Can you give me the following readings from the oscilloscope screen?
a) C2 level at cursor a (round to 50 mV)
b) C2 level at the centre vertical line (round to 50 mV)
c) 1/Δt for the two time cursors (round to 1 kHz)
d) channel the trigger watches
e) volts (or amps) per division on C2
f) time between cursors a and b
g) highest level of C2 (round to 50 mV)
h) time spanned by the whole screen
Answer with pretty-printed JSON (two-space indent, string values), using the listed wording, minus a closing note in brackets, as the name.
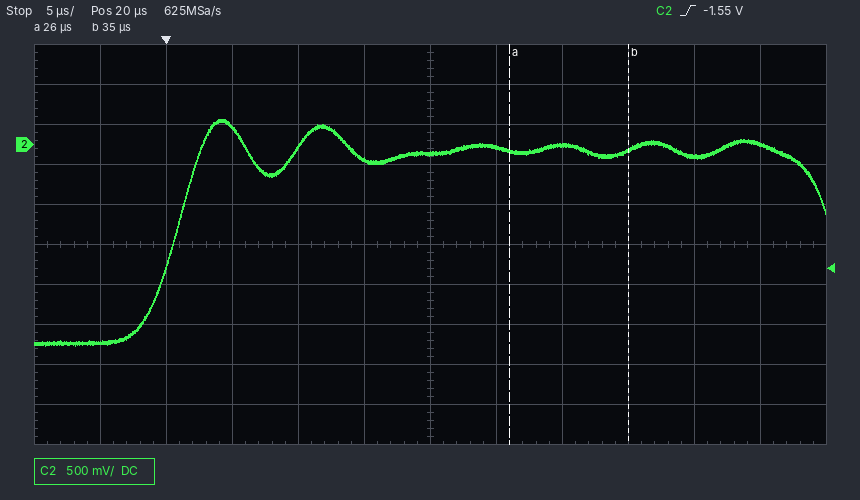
{
  "C2 level at cursor a": "-100 mV",
  "C2 level at the centre vertical line": "-100 mV",
  "1/Δt for the two time cursors": "111 kHz",
  "channel the trigger watches": "C2",
  "volts (or amps) per division on C2": "500 mV",
  "time between cursors a and b": "9.0 µs",
  "highest level of C2": "300 mV",
  "time spanned by the whole screen": "60 µs"
}
